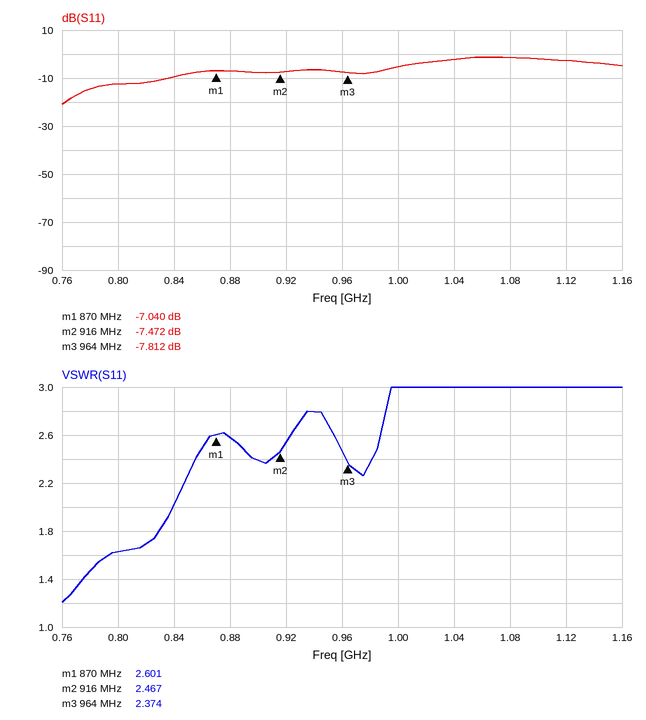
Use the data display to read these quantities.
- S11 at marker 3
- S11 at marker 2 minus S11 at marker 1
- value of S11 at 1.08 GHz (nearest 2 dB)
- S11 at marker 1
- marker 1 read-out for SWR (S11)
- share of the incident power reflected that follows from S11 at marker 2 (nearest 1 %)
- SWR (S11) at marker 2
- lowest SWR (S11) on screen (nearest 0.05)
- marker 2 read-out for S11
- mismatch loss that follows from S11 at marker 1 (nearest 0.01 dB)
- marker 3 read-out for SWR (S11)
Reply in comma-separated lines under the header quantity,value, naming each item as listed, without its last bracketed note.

quantity,value
S11 at marker 3,-7.812 dB
S11 at marker 2 minus S11 at marker 1,-0.432 dB
value of S11 at 1.08 GHz,-2 dB
S11 at marker 1,-7.040 dB
marker 1 read-out for SWR,2.601
share of the incident power reflected that follows from S11 at marker 2,18 %
SWR (S11) at marker 2,2.467
lowest SWR (S11) on screen,1.20
marker 2 read-out for S11,-7.472 dB
mismatch loss that follows from S11 at marker 1,0.96 dB
marker 3 read-out for SWR,2.374
